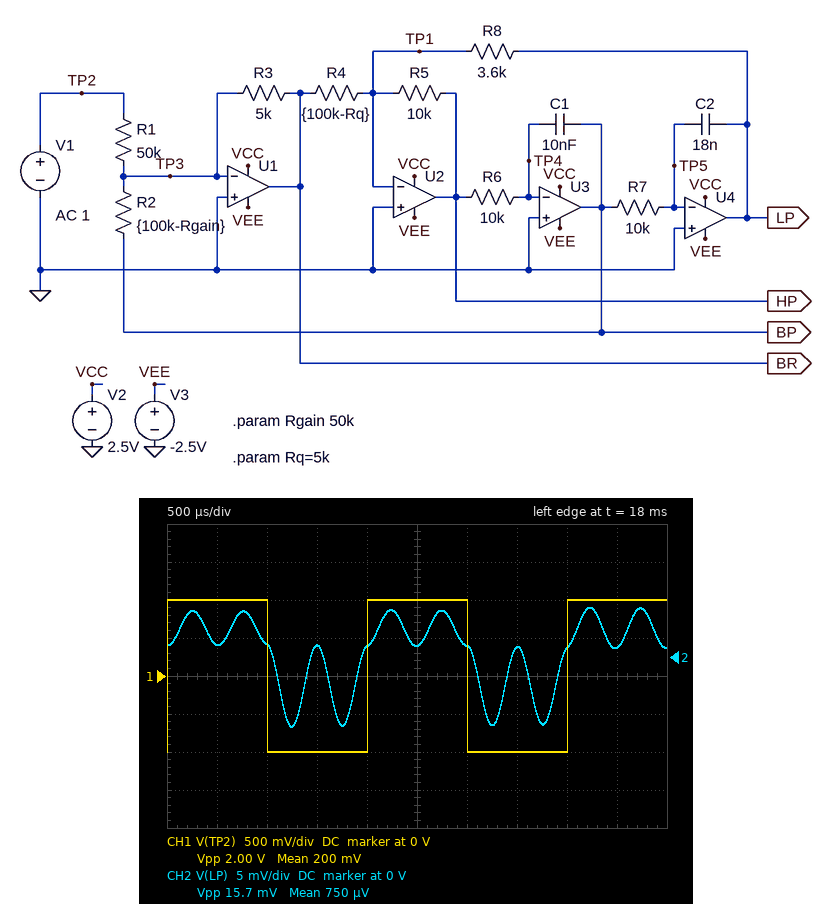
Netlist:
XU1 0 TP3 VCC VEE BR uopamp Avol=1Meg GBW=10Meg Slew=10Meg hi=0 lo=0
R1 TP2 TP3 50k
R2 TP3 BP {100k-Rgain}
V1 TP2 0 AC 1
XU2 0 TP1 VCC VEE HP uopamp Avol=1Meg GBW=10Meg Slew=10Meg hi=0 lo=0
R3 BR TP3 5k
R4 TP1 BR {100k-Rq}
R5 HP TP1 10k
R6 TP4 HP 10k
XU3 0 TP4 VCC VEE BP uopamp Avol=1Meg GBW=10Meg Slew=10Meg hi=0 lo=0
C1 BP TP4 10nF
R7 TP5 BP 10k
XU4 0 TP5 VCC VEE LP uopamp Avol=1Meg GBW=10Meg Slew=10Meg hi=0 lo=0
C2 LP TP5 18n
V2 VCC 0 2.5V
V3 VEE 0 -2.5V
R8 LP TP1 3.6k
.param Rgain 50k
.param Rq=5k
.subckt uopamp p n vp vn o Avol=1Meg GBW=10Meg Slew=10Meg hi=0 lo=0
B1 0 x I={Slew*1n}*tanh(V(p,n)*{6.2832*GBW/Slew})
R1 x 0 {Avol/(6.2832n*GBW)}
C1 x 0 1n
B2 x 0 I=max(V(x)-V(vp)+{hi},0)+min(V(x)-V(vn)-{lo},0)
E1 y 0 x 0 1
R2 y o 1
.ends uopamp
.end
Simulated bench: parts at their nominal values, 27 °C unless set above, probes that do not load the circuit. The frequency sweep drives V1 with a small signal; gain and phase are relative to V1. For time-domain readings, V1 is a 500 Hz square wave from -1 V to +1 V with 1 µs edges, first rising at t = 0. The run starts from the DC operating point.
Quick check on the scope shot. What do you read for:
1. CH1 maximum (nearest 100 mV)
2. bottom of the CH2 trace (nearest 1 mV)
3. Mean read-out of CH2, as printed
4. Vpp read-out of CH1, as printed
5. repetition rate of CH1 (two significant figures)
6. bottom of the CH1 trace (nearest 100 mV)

1.0 V
-9 mV
750 µV
2.00 V
500 Hz
-1.0 V
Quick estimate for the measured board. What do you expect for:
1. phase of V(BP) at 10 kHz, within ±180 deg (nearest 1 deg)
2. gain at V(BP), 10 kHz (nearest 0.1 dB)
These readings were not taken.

90 deg
-55.2 dB
